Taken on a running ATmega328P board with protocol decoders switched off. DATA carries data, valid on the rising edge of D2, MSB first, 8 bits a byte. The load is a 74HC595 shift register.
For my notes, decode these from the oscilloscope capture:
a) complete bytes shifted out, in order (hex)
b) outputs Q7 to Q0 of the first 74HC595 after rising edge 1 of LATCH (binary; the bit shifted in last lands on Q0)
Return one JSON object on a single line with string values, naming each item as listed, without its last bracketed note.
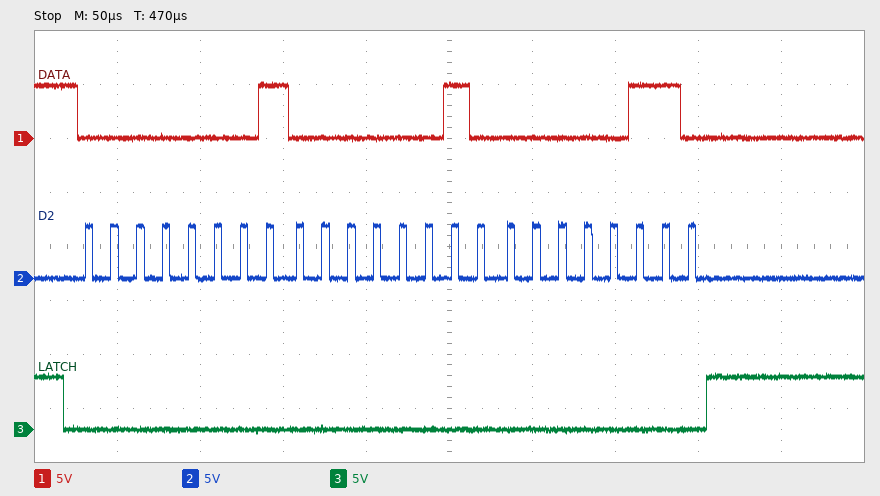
{"complete bytes shifted out, in order": "01 02 06", "outputs Q7 to Q0 of the first 74HC595 after rising edge 1 of LATCH": "00000110"}
